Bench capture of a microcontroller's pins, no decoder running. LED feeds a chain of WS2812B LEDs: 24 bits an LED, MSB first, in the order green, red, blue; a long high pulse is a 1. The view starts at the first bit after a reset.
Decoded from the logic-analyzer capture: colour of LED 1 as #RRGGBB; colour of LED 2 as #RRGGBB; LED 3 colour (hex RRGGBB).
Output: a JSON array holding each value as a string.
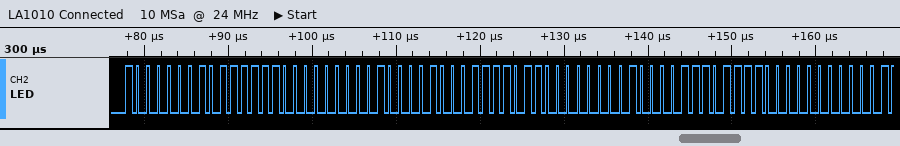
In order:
["#7E8100", "#7B8400", "#788700"]
